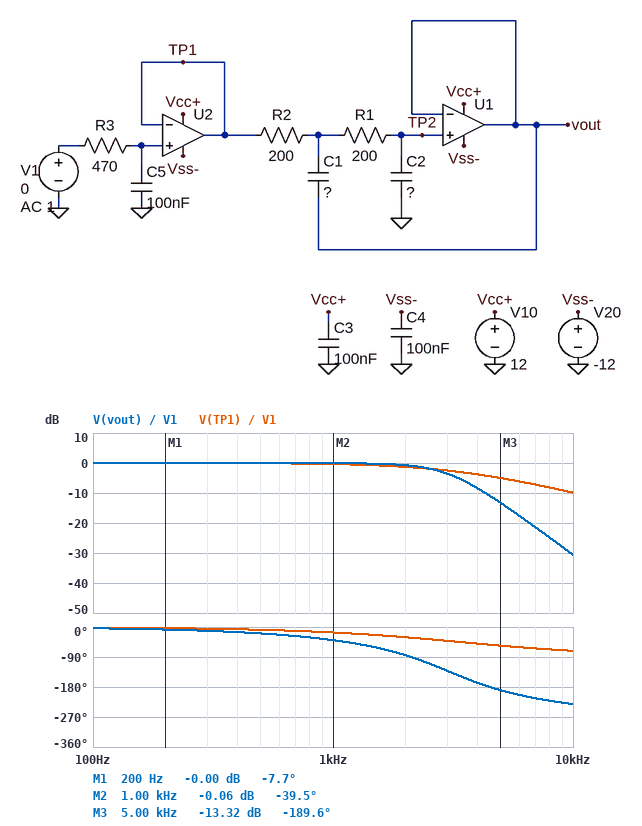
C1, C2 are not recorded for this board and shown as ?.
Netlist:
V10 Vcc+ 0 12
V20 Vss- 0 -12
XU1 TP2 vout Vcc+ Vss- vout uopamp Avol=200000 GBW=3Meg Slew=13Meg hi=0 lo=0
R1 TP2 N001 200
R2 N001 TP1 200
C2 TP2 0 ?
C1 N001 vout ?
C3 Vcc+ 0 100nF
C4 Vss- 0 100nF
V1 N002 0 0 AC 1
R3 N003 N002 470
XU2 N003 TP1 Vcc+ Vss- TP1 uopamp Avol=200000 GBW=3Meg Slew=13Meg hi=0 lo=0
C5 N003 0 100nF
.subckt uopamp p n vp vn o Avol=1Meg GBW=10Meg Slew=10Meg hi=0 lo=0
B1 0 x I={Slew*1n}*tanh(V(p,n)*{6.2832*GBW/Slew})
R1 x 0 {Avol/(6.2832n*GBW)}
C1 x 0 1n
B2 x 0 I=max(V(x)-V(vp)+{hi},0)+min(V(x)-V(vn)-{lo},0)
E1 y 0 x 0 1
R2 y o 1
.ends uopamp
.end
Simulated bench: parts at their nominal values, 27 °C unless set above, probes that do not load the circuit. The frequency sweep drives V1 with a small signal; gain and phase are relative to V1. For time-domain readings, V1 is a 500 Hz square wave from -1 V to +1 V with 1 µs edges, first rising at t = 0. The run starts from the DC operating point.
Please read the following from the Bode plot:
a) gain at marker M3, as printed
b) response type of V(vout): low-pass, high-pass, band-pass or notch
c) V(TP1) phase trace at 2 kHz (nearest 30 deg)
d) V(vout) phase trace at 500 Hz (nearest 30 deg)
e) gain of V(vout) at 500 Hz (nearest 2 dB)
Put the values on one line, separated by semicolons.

-13.32 dB; low-pass; -30 deg; -30 deg; 0 dB
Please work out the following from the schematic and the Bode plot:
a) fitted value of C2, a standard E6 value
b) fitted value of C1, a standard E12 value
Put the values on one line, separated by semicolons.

150 nF; 470 nF
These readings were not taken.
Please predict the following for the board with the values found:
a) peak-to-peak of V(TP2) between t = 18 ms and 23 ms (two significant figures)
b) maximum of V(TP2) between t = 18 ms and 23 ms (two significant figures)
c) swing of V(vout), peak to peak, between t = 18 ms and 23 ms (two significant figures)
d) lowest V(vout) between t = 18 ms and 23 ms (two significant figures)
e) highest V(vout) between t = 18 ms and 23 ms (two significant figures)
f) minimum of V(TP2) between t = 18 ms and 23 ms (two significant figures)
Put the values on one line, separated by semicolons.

2.3 V; 1.1 V; 2.3 V; -1.1 V; 1.1 V; -1.1 V
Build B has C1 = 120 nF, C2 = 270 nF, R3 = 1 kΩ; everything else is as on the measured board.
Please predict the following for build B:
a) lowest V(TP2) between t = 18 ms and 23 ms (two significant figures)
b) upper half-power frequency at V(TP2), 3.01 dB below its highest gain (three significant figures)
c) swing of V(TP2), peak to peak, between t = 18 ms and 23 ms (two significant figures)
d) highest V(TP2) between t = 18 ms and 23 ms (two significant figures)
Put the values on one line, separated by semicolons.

-1.0 V; 1.05 kHz; 2.0 V; 1.0 V
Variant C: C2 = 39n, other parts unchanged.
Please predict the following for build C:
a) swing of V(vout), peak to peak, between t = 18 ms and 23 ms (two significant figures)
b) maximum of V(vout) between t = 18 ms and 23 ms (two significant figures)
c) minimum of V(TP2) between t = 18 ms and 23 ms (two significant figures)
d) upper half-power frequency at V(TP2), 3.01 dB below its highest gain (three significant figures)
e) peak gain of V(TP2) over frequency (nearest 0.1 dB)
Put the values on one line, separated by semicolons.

2.4 V; 1.2 V; -1.2 V; 6.41 kHz; 0 dB
